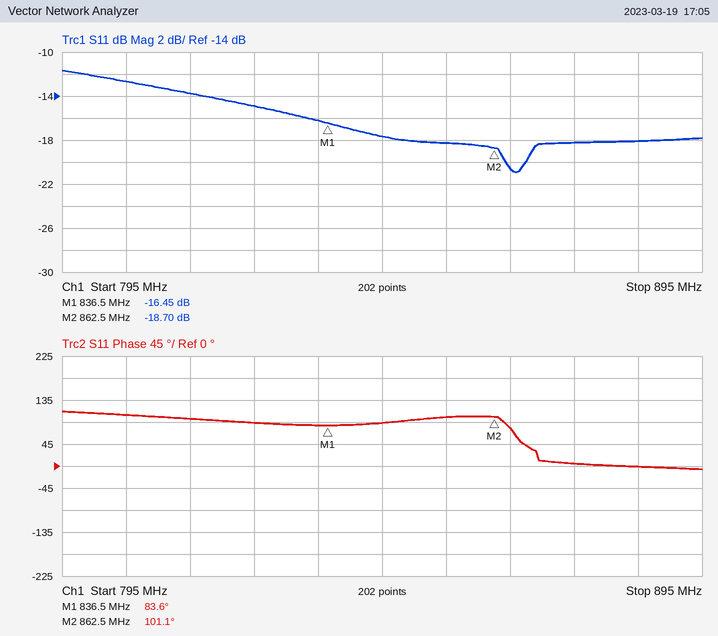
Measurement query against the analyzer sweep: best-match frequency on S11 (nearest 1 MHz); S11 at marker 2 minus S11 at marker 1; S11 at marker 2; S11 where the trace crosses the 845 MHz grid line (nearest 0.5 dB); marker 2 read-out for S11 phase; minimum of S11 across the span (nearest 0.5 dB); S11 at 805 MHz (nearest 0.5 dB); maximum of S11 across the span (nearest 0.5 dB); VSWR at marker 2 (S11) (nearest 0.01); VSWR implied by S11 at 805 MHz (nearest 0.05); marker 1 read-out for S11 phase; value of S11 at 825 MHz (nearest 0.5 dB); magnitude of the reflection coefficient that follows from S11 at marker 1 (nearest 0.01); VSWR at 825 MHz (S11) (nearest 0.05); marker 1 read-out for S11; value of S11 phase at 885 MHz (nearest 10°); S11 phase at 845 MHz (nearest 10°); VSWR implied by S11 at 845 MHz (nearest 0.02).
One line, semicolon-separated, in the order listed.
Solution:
866 MHz; -2.25 dB; -18.70 dB; -17.5 dB; 101.1°; -21.0 dB; -12.5 dB; -11.5 dB; 1.26; 1.60; 83.6°; -15.0 dB; 0.15; 1.45; -16.45 dB; 0°; 90°; 1.30
